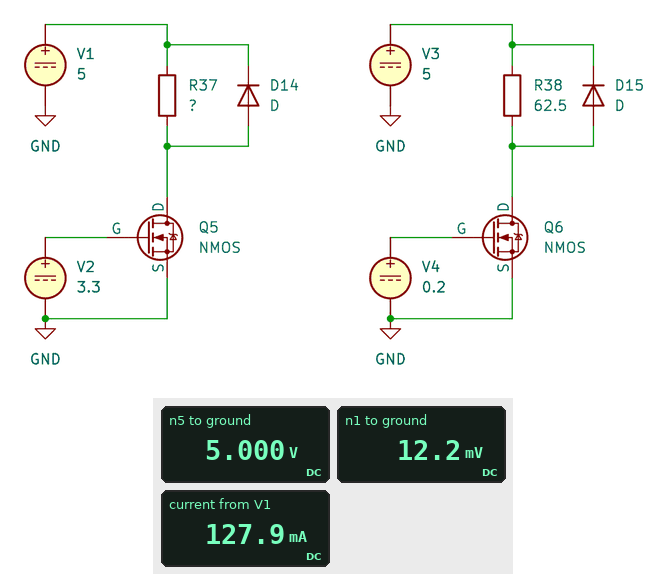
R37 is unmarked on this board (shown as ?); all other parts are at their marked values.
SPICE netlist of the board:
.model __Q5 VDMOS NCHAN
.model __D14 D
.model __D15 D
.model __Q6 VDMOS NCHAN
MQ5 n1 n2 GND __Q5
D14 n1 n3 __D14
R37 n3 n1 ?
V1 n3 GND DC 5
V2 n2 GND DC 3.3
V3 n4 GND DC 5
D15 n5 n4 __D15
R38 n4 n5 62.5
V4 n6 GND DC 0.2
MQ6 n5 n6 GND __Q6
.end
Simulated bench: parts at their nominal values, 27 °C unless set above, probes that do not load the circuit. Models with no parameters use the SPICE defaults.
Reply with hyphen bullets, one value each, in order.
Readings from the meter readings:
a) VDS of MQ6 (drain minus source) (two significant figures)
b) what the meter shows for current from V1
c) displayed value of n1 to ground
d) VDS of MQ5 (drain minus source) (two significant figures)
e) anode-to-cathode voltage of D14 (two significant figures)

- 5.0 V
- 127.9 mA
- 12.2 mV
- 12 mV
- -5.0 V
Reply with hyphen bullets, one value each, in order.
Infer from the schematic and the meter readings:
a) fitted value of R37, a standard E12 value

- 39 Ω
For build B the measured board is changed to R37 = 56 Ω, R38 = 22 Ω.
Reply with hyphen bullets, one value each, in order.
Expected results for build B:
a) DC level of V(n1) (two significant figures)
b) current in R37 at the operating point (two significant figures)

- 8.5 mV
- 89 mA
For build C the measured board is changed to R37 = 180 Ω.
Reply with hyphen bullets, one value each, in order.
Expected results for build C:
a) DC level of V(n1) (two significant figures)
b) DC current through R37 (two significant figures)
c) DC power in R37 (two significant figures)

- 2.6 mV
- 28 mA
- 140 mW
